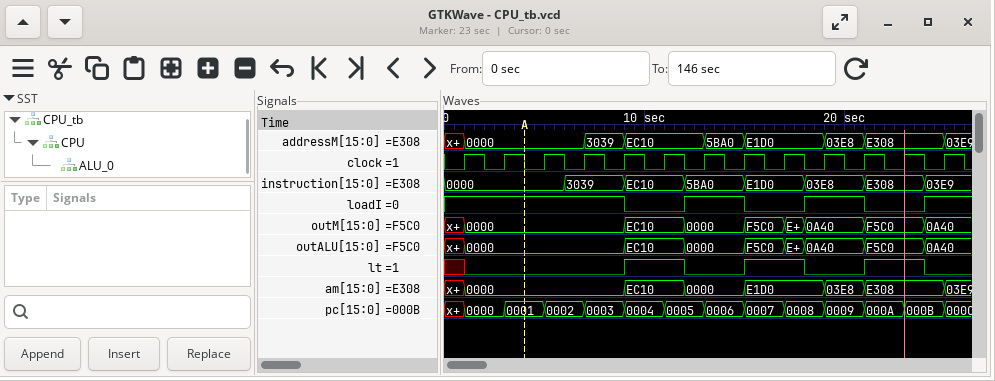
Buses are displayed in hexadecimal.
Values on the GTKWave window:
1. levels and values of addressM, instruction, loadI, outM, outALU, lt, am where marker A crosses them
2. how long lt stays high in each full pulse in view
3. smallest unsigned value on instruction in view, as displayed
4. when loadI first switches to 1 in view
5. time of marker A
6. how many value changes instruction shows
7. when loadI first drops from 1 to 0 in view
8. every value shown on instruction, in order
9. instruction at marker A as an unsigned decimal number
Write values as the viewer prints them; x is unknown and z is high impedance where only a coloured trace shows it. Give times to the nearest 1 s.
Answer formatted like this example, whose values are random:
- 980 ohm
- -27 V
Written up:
- addressM=0000, instruction=0000, loadI=1, outM=0000, outALU=0000, lt=0, am=0000
- 3 s, 3 s, 3 s
- 0000
- 12 s
- 4 s
- 7
- 9 s
- 0000, 3039, EC10, 5BA0, E1D0, 03E8, E308, 03E9
- 0
